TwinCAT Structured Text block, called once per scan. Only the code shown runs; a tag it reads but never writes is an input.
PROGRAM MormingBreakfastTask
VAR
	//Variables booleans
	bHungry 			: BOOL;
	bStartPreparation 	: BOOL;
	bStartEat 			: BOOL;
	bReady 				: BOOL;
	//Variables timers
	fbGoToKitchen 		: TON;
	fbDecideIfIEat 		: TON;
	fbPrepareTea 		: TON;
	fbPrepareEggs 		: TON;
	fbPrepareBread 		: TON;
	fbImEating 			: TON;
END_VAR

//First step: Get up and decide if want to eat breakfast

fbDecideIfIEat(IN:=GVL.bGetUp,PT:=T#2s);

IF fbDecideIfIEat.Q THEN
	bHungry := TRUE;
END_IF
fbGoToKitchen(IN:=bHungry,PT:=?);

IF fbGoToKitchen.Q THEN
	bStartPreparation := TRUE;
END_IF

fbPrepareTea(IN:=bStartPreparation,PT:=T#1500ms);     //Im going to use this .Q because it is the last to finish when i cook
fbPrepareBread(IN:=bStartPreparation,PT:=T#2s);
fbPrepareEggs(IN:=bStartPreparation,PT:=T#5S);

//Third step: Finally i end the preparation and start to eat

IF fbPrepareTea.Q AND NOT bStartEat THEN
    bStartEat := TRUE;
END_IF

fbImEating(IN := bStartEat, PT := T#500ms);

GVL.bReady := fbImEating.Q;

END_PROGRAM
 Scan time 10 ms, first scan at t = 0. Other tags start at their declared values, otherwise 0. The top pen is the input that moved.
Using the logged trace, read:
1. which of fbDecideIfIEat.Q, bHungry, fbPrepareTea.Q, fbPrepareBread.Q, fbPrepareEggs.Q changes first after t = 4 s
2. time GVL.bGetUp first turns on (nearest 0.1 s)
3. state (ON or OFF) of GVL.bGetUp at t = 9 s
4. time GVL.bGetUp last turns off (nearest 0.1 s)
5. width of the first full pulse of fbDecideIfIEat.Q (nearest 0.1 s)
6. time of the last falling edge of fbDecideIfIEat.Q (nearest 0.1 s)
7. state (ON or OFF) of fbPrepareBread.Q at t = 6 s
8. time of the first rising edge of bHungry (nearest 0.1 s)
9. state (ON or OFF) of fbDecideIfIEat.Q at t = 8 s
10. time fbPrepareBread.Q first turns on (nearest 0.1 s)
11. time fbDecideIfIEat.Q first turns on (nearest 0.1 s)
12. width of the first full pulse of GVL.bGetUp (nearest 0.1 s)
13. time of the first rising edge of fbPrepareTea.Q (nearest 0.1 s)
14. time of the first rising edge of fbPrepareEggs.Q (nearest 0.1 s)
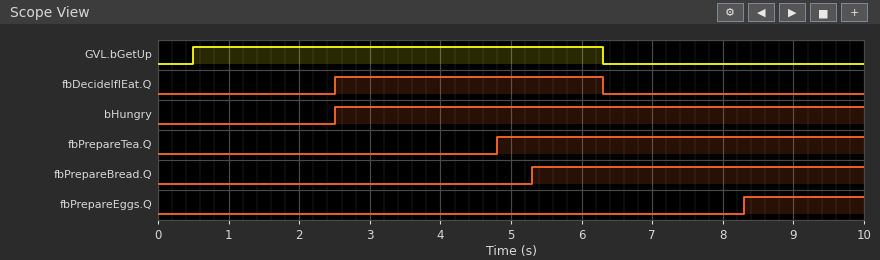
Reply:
fbPrepareTea.Q
0.5 s
OFF
6.3 s
3.8 s
6.3 s
ON
2.5 s
OFF
5.3 s
2.5 s
5.8 s
4.8 s
8.3 s
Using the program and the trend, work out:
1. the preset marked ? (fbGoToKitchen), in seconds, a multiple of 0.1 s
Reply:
0.8 s
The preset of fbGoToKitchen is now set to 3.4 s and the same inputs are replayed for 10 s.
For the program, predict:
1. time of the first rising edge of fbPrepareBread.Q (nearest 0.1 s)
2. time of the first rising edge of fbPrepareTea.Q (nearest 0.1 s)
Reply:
7.9 s
7.4 s
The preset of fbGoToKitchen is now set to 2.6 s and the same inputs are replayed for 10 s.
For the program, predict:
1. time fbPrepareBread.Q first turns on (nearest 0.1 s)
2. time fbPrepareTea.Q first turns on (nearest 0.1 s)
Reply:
7.1 s
6.6 s
